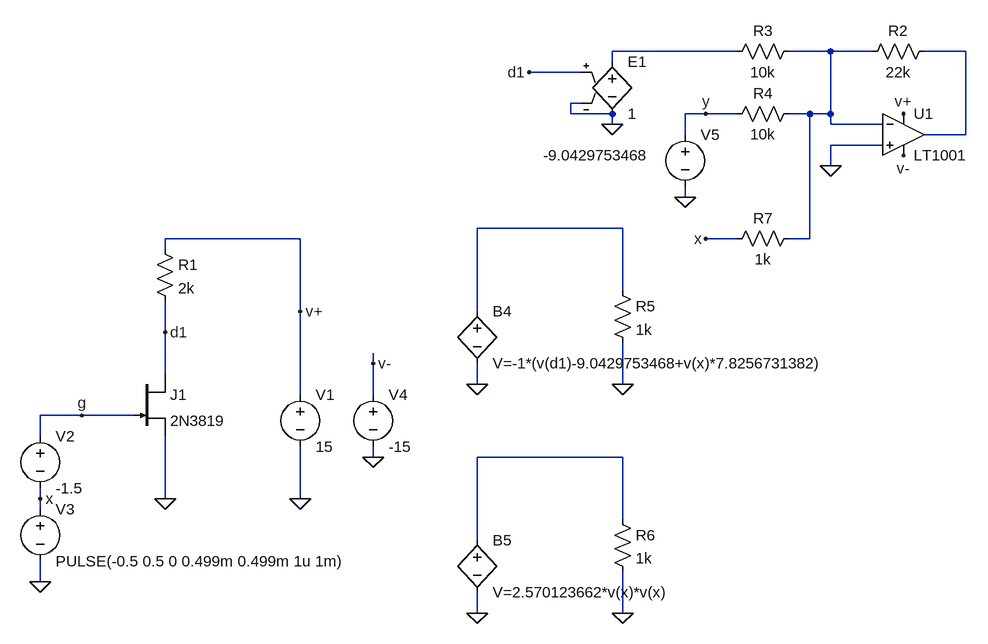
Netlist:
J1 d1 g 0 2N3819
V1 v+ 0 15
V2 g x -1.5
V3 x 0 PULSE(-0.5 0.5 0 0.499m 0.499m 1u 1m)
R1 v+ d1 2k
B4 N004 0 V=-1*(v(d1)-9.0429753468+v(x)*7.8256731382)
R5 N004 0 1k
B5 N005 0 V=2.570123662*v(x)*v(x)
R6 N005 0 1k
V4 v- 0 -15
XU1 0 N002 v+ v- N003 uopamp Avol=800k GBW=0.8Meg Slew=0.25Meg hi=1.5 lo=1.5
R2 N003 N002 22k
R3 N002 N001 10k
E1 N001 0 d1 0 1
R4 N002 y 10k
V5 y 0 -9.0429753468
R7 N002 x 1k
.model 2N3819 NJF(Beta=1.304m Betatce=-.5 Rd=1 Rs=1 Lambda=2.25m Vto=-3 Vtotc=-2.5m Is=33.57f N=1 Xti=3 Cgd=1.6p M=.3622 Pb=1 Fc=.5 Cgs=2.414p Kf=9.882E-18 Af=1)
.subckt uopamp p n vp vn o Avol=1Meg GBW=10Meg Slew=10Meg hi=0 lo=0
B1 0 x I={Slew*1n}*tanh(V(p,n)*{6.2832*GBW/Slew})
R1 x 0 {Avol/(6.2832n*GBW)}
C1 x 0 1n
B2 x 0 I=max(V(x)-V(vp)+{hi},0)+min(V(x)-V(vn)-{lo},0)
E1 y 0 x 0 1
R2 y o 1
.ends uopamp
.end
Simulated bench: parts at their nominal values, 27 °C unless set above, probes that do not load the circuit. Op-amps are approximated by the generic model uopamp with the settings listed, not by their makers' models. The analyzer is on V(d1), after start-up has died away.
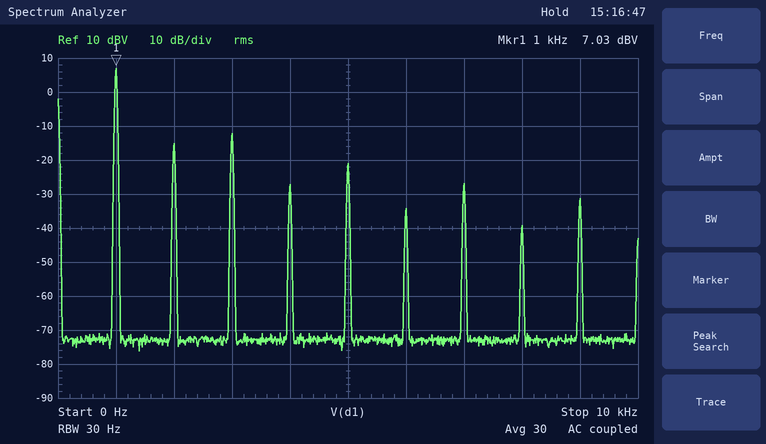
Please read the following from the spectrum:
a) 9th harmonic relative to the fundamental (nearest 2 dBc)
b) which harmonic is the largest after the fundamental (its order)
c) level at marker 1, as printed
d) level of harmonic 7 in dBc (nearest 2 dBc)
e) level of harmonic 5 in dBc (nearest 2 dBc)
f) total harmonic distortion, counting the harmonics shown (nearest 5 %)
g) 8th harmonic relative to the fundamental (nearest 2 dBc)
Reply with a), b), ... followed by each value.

a) -38 dBc
b) 3
c) 7.03 dBV
d) -34 dBc
e) -28 dBc
f) 15 %
g) -46 dBc
